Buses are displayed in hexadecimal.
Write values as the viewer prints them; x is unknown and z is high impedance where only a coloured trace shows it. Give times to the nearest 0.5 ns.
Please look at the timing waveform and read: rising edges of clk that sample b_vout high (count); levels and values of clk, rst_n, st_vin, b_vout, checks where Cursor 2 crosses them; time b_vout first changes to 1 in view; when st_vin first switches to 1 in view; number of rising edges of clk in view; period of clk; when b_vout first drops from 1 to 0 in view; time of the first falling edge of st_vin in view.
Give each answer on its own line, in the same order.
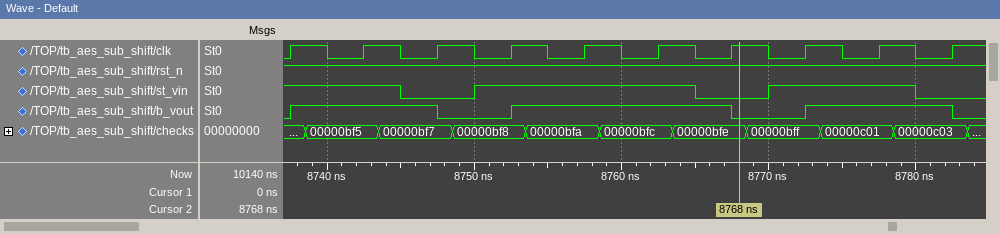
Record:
7
clk=1, rst_n=1, st_vin=0, b_vout=0, checks=00000bfe
8737.5 ns
8750 ns
10
5 ns
8747.5 ns
8745 ns
